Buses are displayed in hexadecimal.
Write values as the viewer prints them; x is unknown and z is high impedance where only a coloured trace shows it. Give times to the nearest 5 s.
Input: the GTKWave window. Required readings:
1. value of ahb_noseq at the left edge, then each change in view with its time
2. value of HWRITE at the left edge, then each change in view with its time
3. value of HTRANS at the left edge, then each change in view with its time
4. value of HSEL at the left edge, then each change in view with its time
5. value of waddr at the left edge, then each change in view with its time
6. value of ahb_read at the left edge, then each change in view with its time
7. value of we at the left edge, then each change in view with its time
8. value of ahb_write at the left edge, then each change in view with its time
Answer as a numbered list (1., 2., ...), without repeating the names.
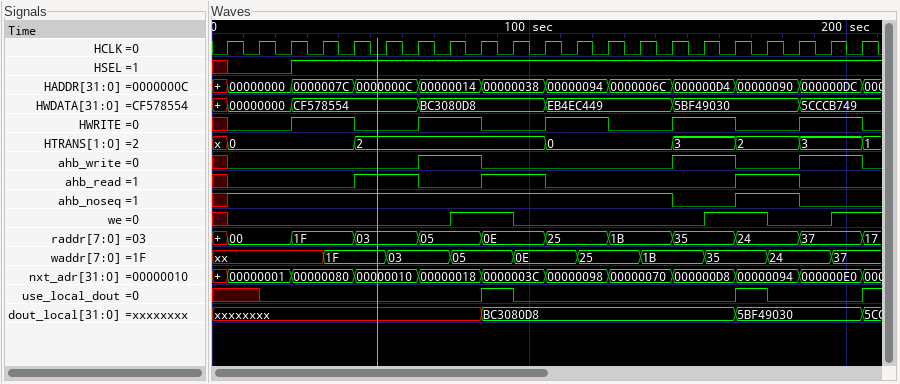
1. x, 1 at 5 s, 0 at 145 s, 1 at 165 s, 0 at 185 s
2. x, 0 at 5 s, 1 at 25 s, 0 at 45 s, 1 at 65 s, 0 at 85 s, 1 at 105 s, 0 at 125 s, 1 at 145 s, 0 at 165 s, 1 at 185 s, 0 at 205 s
3. x, 0 at 5 s, 2 at 45 s, 0 at 105 s, 3 at 145 s, 2 at 165 s, 3 at 185 s, 1 at 205 s
4. x, 0 at 5 s, 1 at 25 s
5. xx, 1F at 35 s, 03 at 55 s, 05 at 75 s, 0E at 95 s, 25 at 115 s, 1B at 135 s, 35 at 155 s, 24 at 175 s, 37 at 195 s
6. x, 0 at 5 s, 1 at 45 s, 0 at 65 s, 1 at 85 s, 0 at 105 s, 1 at 165 s, 0 at 185 s
7. x, 0 at 5 s, 1 at 75 s, 0 at 95 s, 1 at 155 s, 0 at 175 s, 1 at 195 s
8. x, 0 at 5 s, 1 at 65 s, 0 at 85 s, 1 at 145 s, 0 at 165 s, 1 at 185 s, 0 at 205 s
